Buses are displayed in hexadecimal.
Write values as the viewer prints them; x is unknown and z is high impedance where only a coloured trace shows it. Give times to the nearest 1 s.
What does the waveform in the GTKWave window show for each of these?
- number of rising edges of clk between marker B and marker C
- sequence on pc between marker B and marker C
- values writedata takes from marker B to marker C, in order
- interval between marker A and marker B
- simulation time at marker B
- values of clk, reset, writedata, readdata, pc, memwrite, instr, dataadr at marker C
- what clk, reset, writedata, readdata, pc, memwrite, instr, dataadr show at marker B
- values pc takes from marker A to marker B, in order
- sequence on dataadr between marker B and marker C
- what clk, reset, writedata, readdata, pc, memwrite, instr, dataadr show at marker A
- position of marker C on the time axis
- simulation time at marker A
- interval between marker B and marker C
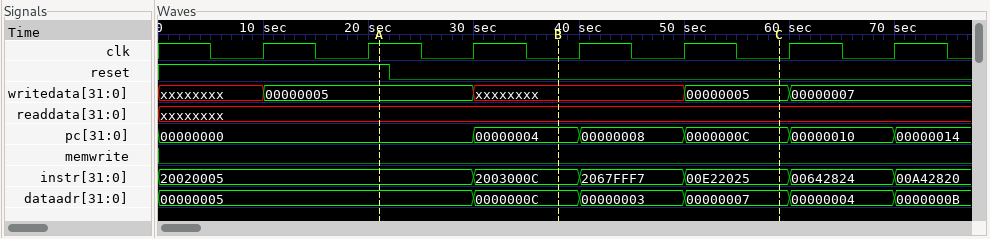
2
00000004, 00000008, 0000000C
xxxxxxxx, 00000005
17 s
38 s
clk=0, reset=0, writedata=00000005, readdata=xxxxxxxx, pc=0000000C, memwrite=0, instr=00E22025, dataadr=00000007
clk=0, reset=0, writedata=xxxxxxxx, readdata=xxxxxxxx, pc=00000004, memwrite=0, instr=2003000C, dataadr=0000000C
00000000, 00000004
0000000C, 00000003, 00000007
clk=1, reset=1, writedata=00000005, readdata=xxxxxxxx, pc=00000000, memwrite=0, instr=20020005, dataadr=00000005
59 s
21 s
21 s
